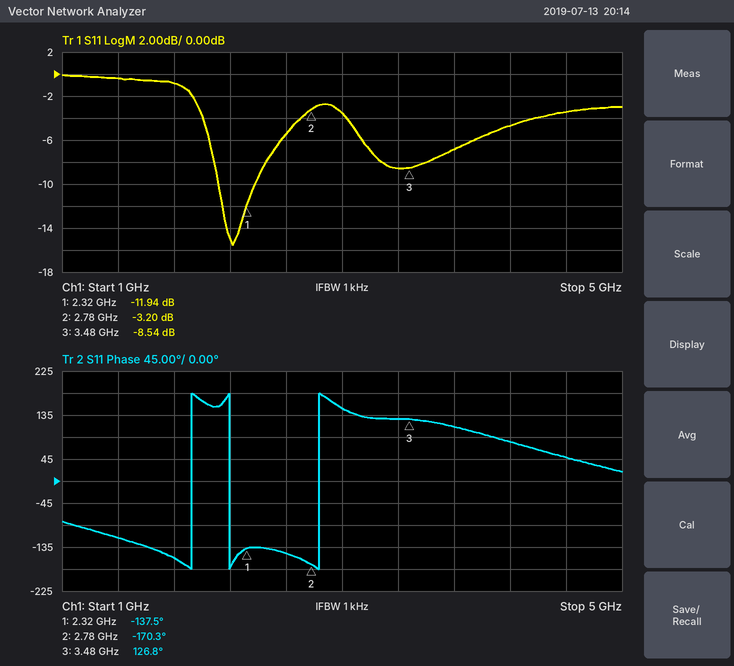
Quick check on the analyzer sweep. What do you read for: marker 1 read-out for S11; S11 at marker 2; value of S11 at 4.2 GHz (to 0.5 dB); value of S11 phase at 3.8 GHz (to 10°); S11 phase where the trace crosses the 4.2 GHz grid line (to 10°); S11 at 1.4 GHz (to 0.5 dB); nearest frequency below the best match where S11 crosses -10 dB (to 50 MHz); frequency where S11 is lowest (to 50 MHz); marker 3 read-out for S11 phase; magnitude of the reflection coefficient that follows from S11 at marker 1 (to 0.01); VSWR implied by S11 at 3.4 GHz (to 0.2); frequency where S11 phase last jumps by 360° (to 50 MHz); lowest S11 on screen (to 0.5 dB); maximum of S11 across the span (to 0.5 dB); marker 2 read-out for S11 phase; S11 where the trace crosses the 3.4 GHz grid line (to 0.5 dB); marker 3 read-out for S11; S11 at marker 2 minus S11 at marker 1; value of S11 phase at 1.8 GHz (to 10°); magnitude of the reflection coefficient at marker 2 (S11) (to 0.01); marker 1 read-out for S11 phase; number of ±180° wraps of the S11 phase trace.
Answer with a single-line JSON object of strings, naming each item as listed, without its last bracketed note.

{"marker 1 read-out for S11": "-11.94 dB", "S11 at marker 2": "-3.20 dB", "value of S11 at 4.2 GHz": "-4.5 dB", "value of S11 phase at 3.8 GHz": "110°", "S11 phase where the trace crosses the 4.2 GHz grid line": "80°", "S11 at 1.4 GHz": "-0.5 dB", "nearest frequency below the best match where S11 crosses -10 dB": "2.10 GHz", "frequency where S11 is lowest": "2.20 GHz", "marker 3 read-out for S11 phase": "126.8°", "magnitude of the reflection coefficient that follows from S11 at marker 1": "0.25", "VSWR implied by S11 at 3.4 GHz": "2.2", "frequency where S11 phase last jumps by 360°": "2.85 GHz", "lowest S11 on screen": "-15.5 dB", "maximum of S11 across the span": "0.0 dB", "marker 2 read-out for S11 phase": "-170.3°", "S11 where the trace crosses the 3.4 GHz grid line": "-8.5 dB", "marker 3 read-out for S11": "-8.54 dB", "S11 at marker 2 minus S11 at marker 1": "8.74 dB", "value of S11 phase at 1.8 GHz": "-160°", "magnitude of the reflection coefficient at marker 2 (S11)": "0.69", "marker 1 read-out for S11 phase": "-137.5°", "number of ±180° wraps of the S11 phase trace": "3"}
